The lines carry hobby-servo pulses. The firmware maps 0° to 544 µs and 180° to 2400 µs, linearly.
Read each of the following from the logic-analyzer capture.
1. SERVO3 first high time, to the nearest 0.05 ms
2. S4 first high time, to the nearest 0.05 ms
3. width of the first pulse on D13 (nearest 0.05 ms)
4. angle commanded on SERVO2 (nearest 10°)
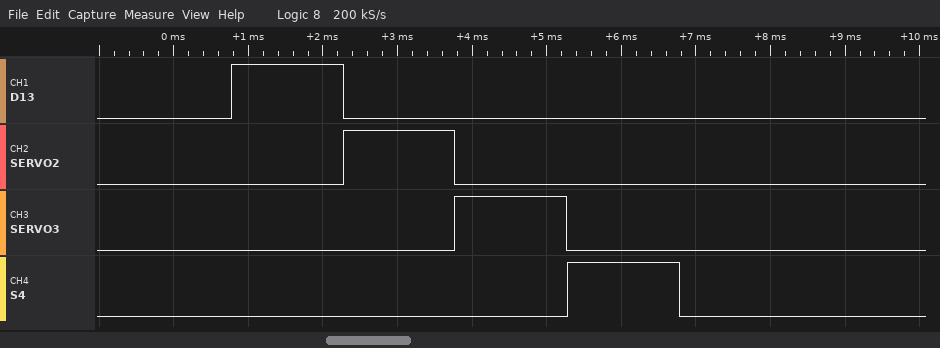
1.50 ms
1.50 ms
1.50 ms
90°
